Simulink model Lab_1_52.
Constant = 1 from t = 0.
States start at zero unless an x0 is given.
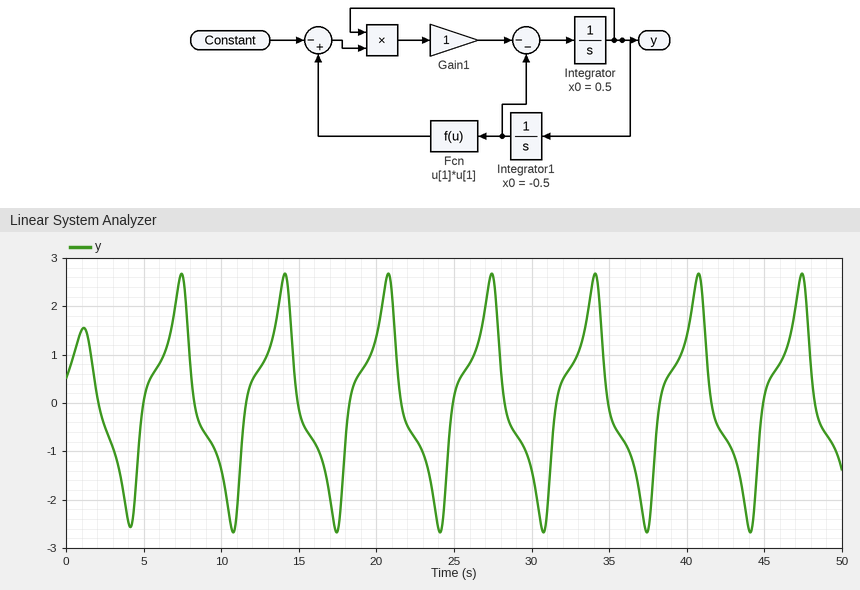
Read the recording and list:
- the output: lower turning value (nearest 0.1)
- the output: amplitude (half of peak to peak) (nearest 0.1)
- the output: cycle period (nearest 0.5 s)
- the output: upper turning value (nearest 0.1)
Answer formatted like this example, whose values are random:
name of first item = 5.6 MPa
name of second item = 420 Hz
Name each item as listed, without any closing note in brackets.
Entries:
the output: lower turning value = -2.7
the output: amplitude (half of peak to peak) = 2.7
the output: cycle period = 6.5 s
the output: upper turning value = 2.7
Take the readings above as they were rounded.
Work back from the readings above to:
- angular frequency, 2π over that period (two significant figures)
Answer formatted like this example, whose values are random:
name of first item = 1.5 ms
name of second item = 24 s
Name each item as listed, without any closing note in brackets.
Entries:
angular frequency, 2π over that period = 0.97 rad/s
